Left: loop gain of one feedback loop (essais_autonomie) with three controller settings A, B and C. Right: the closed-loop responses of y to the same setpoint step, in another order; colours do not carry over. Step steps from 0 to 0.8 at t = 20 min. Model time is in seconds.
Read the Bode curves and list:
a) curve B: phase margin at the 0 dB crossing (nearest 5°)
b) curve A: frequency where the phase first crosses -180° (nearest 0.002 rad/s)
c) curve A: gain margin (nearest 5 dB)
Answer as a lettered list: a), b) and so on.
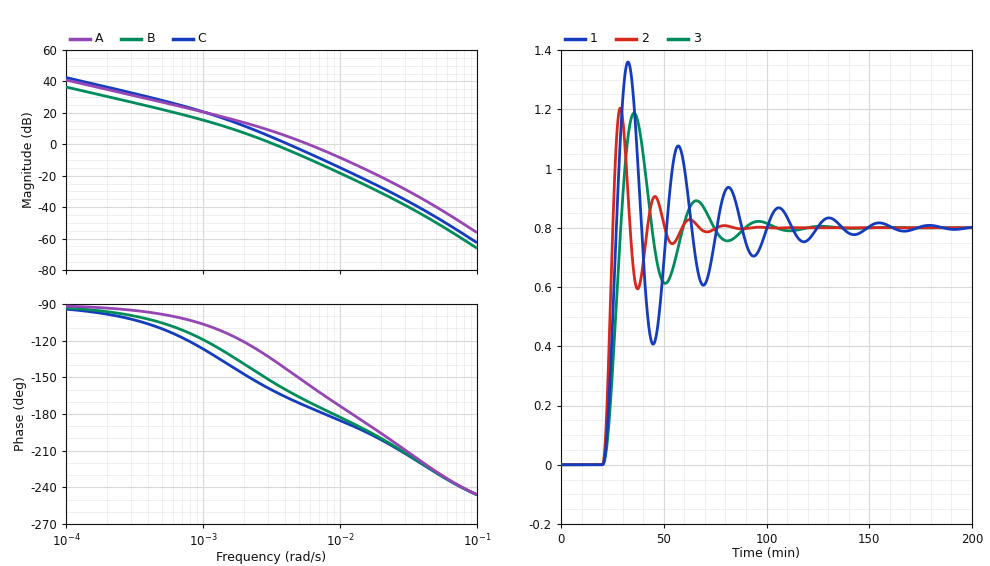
a) 25°
b) 0.012 rad/s
c) 10 dB
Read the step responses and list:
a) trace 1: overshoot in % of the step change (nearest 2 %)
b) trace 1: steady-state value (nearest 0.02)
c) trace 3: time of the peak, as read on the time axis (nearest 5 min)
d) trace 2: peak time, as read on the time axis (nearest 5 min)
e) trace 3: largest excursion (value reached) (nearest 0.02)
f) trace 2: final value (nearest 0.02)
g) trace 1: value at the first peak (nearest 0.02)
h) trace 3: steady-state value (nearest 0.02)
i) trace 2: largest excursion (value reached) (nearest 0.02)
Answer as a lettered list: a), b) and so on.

a) 70 %
b) 0.80
c) 35 min
d) 30 min
e) 1.18
f) 0.80
g) 1.36
h) 0.80
i) 1.20
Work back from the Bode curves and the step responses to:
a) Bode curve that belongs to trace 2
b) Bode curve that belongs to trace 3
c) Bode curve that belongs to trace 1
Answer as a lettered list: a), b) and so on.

a) A
b) B
c) C
